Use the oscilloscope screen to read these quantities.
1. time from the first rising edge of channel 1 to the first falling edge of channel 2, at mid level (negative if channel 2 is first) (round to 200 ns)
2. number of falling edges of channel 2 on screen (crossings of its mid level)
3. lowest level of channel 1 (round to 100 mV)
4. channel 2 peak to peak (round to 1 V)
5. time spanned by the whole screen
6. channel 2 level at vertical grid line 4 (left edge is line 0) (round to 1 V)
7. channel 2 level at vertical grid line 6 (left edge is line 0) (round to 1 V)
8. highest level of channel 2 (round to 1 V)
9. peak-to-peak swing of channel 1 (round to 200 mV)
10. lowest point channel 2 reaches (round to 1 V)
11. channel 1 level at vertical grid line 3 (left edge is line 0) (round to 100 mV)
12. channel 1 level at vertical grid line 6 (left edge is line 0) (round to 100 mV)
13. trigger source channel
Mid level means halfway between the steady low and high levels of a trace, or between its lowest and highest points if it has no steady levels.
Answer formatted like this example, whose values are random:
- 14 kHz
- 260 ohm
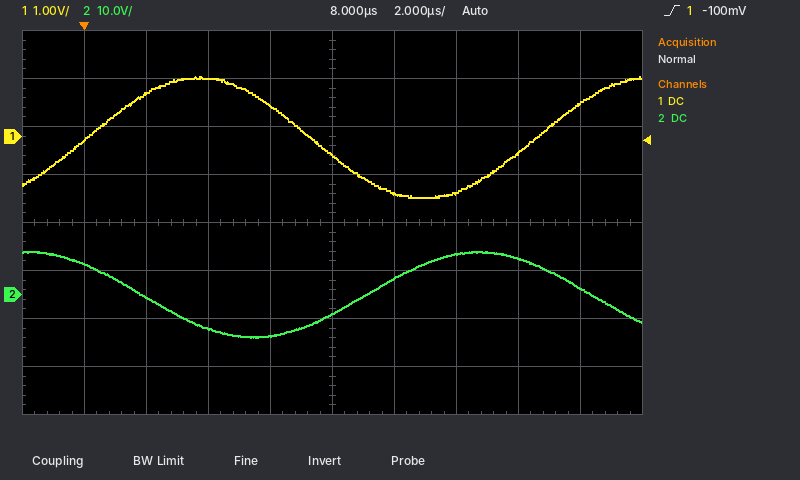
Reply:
- +1.8 µs
- 2
- -1.3 V
- 18 V
- 20 µs
- -9 V
- 3 V
- 9 V
- 2.6 V
- -9 V
- 1.2 V
- -1.2 V
- channel 1
